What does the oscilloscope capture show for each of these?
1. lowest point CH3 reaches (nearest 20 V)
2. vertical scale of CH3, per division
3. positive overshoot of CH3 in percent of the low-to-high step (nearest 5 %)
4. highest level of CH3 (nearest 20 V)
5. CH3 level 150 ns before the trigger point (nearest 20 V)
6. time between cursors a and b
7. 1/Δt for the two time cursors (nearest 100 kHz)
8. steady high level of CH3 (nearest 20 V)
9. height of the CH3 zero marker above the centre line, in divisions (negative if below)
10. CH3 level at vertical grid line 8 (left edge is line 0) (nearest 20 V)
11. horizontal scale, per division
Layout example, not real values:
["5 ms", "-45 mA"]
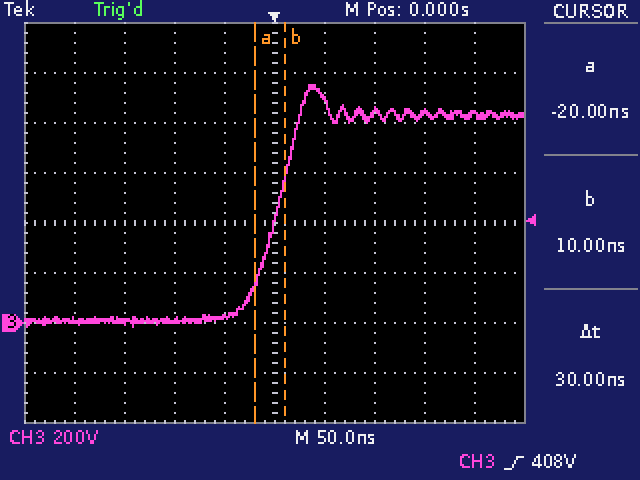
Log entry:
["-20 V", "200 V", "15 %", "960 V", "0 V", "30 ns", "33.3 MHz", "840 V", "-2.0 div", "840 V", "50 ns"]
